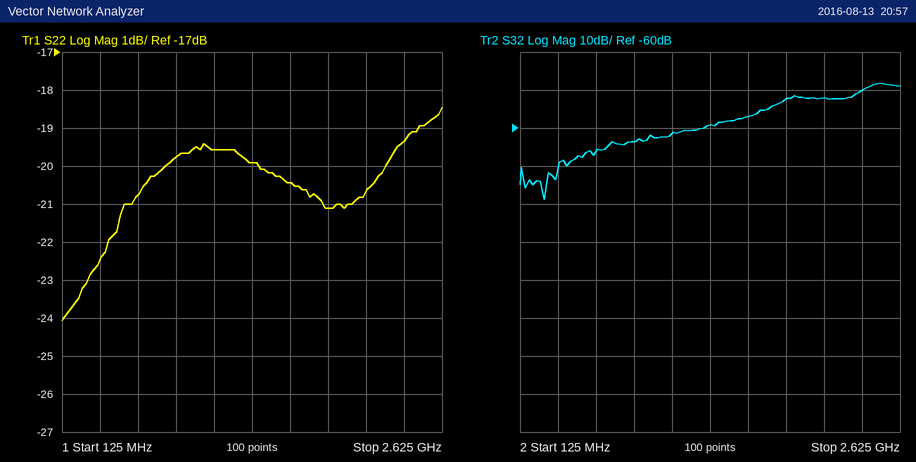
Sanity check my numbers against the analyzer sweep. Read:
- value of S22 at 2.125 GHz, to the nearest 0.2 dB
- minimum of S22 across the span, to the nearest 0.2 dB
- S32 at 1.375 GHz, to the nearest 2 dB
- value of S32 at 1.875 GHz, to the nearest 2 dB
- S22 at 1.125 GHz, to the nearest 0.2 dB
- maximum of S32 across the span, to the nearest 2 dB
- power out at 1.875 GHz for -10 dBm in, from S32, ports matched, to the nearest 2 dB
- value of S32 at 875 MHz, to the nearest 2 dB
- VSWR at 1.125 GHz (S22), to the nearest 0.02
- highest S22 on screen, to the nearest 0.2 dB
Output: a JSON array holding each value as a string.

["-20.6 dB", "-24.0 dB", "-60 dB", "-52 dB", "-19.6 dB", "-48 dB", "-62 dBm", "-64 dB", "1.24", "-18.4 dB"]
